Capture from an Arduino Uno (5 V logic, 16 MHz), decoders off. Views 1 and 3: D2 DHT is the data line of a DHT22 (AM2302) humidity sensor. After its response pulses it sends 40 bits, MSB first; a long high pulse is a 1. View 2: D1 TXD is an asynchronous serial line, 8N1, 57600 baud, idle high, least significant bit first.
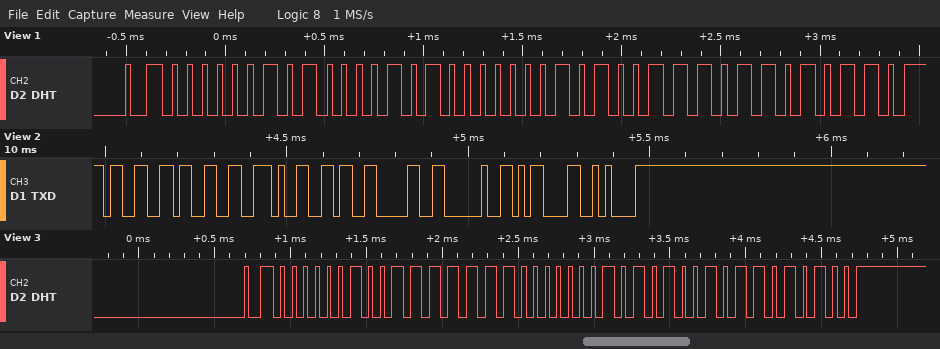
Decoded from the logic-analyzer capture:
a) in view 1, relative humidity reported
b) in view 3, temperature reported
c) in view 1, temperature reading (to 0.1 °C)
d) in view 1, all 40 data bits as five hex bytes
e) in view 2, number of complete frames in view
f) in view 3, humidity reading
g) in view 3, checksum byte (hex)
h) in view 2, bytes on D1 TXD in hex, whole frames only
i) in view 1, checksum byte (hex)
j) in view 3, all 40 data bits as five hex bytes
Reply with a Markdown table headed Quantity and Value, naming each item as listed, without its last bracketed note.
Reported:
| Quantity | Value |
|---|---|
| in view 1, relative humidity reported | 64.5 % |
| in view 3, temperature reported | 33.8 °C |
| in view 1, temperature reading | 33.4 °C |
| in view 1, all 40 data bits as five hex bytes | 02 85 01 4E D6 |
| in view 2, number of complete frames in view | 8 |
| in view 3, humidity reading | 63.9 % |
| in view 3, checksum byte | 0xD4 |
| in view 2, bytes on D1 TXD in hex, whole frames only | 33 33 2E 36 30 20 0D 0A |
| in view 1, checksum byte | 0xD6 |
| in view 3, all 40 data bits as five hex bytes | 02 7F 01 52 D4 |
